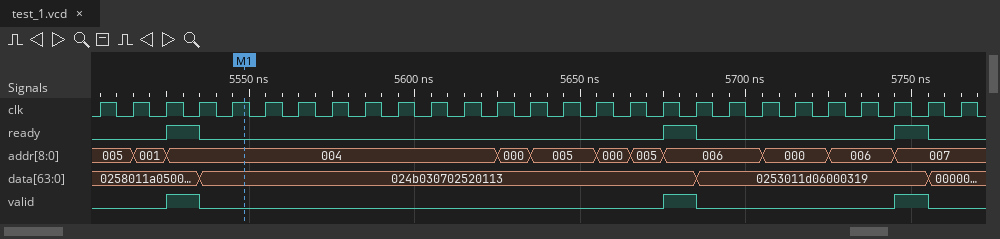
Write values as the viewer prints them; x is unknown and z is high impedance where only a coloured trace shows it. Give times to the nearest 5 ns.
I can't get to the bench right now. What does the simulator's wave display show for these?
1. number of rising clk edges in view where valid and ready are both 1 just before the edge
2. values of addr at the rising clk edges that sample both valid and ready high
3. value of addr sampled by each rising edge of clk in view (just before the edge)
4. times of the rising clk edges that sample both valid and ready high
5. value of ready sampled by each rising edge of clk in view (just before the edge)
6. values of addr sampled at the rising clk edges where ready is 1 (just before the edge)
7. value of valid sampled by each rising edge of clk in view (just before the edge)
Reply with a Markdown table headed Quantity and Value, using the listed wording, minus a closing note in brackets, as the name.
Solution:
| Quantity | Value |
|---|---|
| number of rising clk edges in view where valid and ready are both 1 just before the edge | 3 |
| values of addr at the rising clk edges that sample both valid and ready high | 004, 006, 007 |
| value of addr sampled by each rising edge of clk in view | 005, 005, 001, 004, 004, 004, 004, 004, 004, 004, 004, 004, 004, 000, 005, 005, 000, 005, 006, 006, 006, 000, 000, 006, 006, 007, 007 |
| times of the rising clk edges that sample both valid and ready high | 5535 ns, 5685 ns, 5755 ns |
| value of ready sampled by each rising edge of clk in view | 0 0 0 1 0 0 0 0 0 0 0 0 0 0 0 0 0 0 1 0 0 0 0 0 0 1 0 |
| values of addr sampled at the rising clk edges where ready is 1 | 004, 006, 007 |
| value of valid sampled by each rising edge of clk in view | 0 0 0 1 0 0 0 0 0 0 0 0 0 0 0 0 0 0 1 0 0 0 0 0 0 1 0 |
